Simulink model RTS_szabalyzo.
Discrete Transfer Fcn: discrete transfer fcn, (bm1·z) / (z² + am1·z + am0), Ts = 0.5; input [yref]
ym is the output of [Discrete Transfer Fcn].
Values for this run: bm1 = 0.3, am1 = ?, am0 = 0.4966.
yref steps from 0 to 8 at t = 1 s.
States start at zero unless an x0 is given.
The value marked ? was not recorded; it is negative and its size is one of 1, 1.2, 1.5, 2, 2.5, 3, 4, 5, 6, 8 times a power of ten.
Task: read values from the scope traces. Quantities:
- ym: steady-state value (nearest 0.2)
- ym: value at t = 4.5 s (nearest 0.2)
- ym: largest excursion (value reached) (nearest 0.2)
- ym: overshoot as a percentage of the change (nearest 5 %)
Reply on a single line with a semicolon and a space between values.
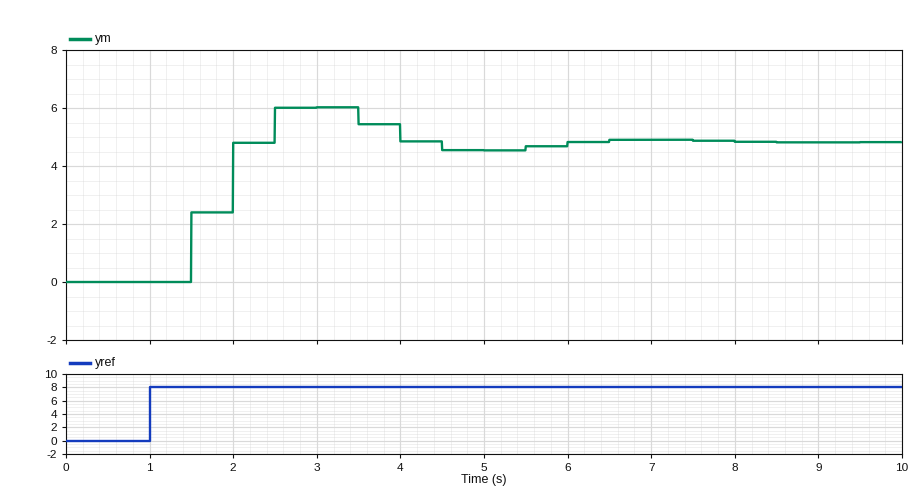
4.8; 4.6; 6.0; 25 %
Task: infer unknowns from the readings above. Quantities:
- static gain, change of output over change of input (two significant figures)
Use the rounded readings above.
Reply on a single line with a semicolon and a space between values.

0.60
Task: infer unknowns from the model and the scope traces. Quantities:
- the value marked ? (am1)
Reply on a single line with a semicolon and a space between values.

-1
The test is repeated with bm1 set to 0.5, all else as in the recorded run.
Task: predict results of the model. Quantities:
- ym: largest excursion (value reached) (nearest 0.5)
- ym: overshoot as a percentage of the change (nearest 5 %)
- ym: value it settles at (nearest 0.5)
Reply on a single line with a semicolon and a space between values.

10.0; 25 %; 8.0
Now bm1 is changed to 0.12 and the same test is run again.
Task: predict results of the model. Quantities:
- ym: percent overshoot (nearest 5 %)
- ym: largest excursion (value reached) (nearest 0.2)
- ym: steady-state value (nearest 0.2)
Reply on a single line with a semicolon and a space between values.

25 %; 2.4; 2.0
